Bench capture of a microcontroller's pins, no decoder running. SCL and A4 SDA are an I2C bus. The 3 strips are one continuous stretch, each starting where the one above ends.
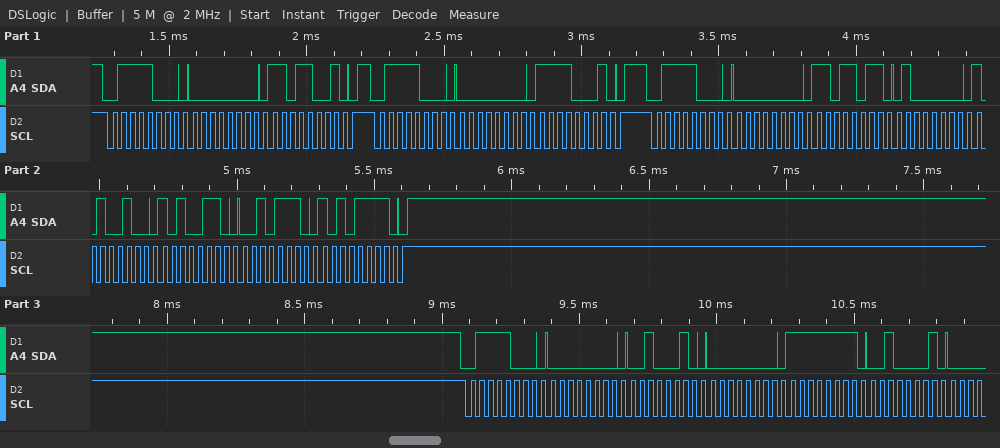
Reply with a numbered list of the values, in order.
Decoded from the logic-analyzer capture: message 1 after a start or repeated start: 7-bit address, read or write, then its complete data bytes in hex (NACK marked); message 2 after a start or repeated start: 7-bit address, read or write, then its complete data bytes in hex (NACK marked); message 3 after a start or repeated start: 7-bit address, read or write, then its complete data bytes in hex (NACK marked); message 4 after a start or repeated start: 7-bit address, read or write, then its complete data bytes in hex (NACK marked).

1. 0x3C write: 00 D9
2. 0x3C write: 00 F1
3. 0x3C write: 00 DB 40 A4 A6 2E AF
4. 0x3C write: 00 22 00 FF 21
